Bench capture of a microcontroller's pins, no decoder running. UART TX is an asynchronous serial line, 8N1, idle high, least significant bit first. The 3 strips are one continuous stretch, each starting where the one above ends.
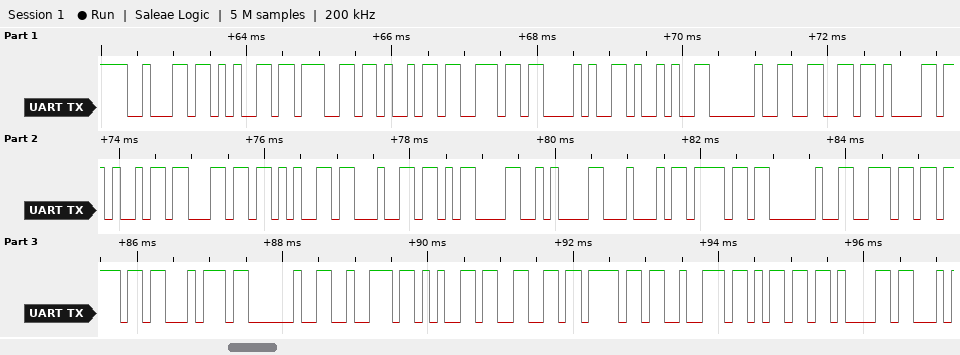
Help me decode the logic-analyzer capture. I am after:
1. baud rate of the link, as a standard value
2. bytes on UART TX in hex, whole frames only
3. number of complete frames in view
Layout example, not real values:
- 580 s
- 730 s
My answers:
- 9600 baud
- 62 65 67 69 6E 28 29 20 66 61 69 6C 65 64 0D 0A 44 6F 20 6E 6F 74 20 72 65 66 6F 72 6D 61
- 30
